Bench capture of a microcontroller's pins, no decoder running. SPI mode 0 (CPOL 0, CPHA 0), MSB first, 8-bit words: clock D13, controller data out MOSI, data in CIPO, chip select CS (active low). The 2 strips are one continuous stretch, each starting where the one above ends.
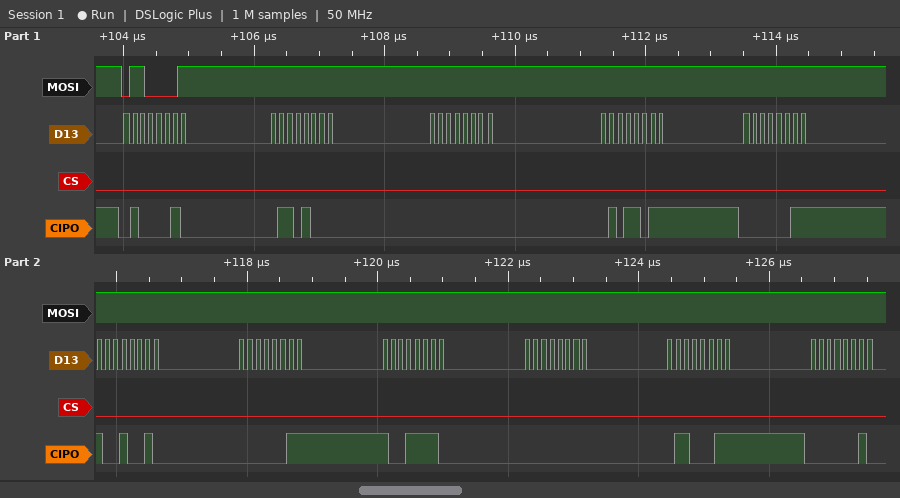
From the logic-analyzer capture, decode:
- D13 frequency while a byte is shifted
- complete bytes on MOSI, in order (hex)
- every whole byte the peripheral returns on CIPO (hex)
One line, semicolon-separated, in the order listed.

8 MHz; 61 FF FF FF FF FF FF FF FF FF FF; 42 68 00 5B 03 92 03 9E 00 63 02
